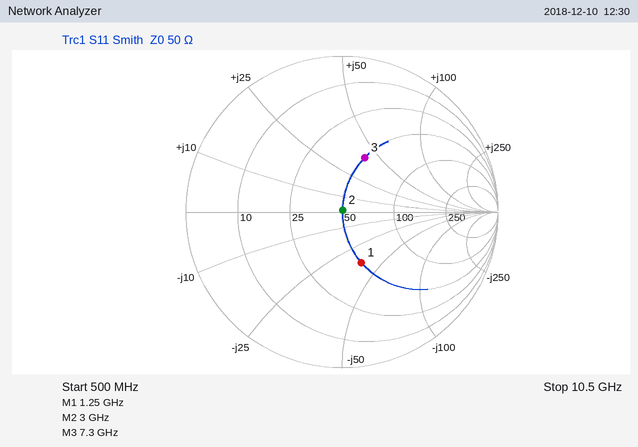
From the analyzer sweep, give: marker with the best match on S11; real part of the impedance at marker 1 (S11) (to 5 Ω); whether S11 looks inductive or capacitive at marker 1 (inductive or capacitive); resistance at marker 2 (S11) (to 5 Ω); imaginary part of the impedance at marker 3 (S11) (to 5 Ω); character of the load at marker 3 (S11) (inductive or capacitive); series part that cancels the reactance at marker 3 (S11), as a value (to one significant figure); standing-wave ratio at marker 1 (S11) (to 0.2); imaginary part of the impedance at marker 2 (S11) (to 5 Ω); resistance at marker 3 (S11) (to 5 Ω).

marker 2
50 Ω
capacitive
50 Ω
+40 Ω
inductive
500 fF
2.0
0 Ω
50 Ω
